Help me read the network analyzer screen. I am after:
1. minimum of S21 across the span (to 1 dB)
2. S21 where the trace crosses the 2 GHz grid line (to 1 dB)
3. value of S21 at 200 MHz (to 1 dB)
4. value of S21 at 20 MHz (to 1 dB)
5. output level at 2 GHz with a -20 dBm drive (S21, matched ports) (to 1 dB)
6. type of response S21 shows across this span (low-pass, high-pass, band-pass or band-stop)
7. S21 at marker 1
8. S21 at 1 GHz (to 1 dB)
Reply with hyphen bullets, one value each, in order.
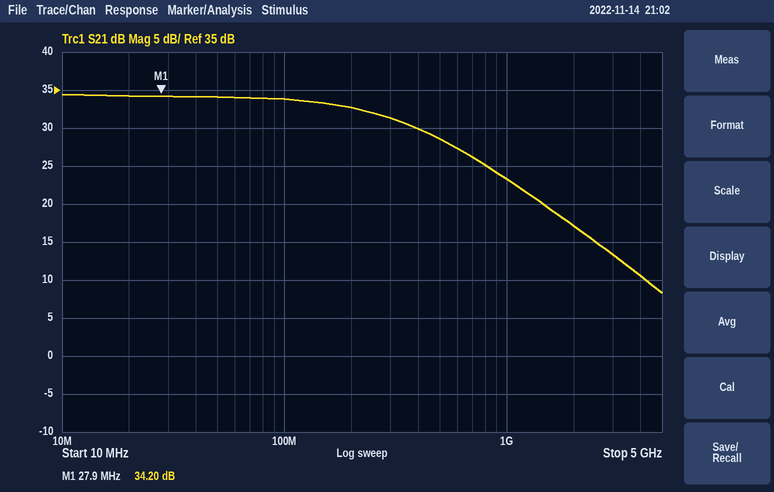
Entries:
- 8 dB
- 17 dB
- 33 dB
- 34 dB
- -3 dBm
- low-pass
- 34.20 dB
- 23 dB
